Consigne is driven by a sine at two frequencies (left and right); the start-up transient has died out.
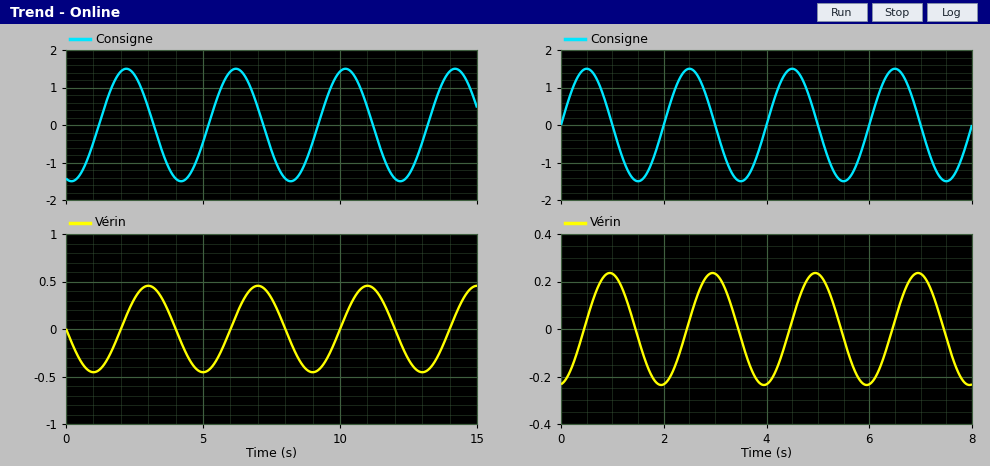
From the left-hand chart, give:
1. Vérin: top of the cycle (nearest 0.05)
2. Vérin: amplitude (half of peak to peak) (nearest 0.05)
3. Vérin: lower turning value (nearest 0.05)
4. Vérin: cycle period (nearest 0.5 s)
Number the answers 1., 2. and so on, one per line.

1. 0.45
2. 0.45
3. -0.45
4. 4.0 s
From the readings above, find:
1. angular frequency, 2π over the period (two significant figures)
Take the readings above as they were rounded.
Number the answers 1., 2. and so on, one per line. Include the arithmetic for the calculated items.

1. 2π / 4 = 1.6 rad/s
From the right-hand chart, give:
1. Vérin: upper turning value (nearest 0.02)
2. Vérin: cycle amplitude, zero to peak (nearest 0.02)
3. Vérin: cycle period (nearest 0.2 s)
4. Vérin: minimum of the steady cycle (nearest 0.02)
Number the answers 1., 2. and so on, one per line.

1. 0.24
2. 0.24
3. 2.0 s
4. -0.24
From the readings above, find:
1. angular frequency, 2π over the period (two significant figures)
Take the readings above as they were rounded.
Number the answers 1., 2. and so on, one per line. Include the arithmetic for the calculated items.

1. 2π / 2 = 3.1 rad/s
